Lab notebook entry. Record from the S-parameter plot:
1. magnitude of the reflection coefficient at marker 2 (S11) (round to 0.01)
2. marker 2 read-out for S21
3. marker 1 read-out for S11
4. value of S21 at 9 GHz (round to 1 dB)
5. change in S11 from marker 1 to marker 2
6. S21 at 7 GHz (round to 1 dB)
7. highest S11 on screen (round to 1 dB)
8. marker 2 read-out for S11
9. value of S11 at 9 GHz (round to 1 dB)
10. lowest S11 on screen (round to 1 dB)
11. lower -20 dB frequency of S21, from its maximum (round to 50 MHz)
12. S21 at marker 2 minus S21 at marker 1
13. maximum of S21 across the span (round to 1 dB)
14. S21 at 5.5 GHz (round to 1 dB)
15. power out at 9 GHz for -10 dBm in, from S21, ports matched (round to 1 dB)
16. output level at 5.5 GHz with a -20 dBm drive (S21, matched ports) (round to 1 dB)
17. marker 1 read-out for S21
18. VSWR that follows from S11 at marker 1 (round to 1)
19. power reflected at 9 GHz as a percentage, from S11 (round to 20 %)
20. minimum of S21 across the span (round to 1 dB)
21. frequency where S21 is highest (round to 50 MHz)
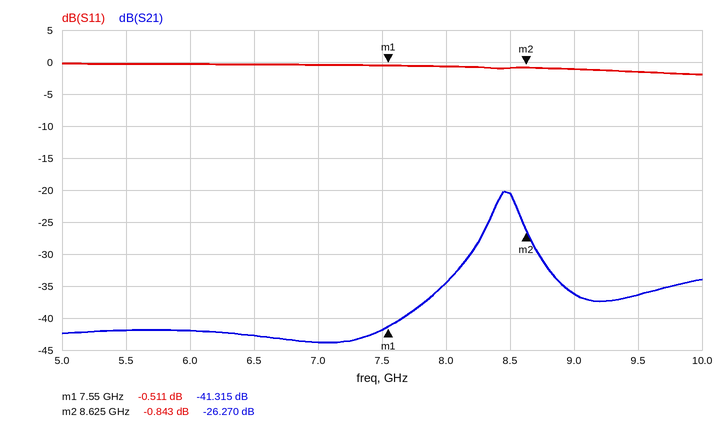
0.91
-26.270 dB
-0.511 dB
-36 dB
-0.332 dB
-44 dB
0 dB
-0.843 dB
-1 dB
-2 dB
7.65 GHz
15.045 dB
-20 dB
-42 dB
-46 dBm
-62 dBm
-41.315 dB
34
80 %
-44 dB
8.45 GHz
